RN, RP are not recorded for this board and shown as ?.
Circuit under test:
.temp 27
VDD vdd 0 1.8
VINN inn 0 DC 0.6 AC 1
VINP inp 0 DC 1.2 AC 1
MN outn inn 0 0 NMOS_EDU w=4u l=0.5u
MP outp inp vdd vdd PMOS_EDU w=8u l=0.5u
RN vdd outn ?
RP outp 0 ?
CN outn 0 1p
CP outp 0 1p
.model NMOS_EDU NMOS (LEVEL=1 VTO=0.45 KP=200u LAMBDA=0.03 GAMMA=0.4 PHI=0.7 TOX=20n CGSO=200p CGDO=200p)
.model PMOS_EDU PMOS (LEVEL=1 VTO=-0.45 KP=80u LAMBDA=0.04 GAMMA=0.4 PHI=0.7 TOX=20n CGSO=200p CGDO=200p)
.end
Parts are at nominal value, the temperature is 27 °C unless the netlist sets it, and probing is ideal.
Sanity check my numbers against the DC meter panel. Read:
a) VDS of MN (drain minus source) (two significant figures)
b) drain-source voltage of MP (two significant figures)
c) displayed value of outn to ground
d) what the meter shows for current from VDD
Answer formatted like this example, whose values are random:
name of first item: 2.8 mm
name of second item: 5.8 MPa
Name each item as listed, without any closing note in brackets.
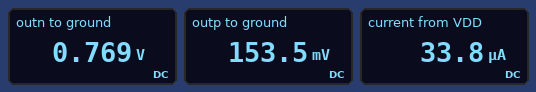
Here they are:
VDS of MN (drain minus source): 770 mV
drain-source voltage of MP: -1.6 V
displayed value of outn to ground: 0.769 V
what the meter shows for current from VDD: 33.8 µA
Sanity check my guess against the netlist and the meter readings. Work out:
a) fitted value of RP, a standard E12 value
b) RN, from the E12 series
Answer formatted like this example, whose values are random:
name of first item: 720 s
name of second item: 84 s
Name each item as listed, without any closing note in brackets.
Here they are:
fitted value of RP, a standard E12 value: 10 kΩ
RN, from the E12 series: 56 kΩ
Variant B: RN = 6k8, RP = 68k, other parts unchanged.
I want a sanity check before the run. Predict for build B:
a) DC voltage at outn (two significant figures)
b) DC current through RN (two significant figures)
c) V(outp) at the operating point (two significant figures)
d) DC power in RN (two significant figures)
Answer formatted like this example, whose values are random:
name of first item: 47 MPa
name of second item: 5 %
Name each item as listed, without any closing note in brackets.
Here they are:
DC voltage at outn: 1.7 V
DC current through RN: 19 µA
V(outp) at the operating point: 1.0 V
DC power in RN: 2.4 µW
